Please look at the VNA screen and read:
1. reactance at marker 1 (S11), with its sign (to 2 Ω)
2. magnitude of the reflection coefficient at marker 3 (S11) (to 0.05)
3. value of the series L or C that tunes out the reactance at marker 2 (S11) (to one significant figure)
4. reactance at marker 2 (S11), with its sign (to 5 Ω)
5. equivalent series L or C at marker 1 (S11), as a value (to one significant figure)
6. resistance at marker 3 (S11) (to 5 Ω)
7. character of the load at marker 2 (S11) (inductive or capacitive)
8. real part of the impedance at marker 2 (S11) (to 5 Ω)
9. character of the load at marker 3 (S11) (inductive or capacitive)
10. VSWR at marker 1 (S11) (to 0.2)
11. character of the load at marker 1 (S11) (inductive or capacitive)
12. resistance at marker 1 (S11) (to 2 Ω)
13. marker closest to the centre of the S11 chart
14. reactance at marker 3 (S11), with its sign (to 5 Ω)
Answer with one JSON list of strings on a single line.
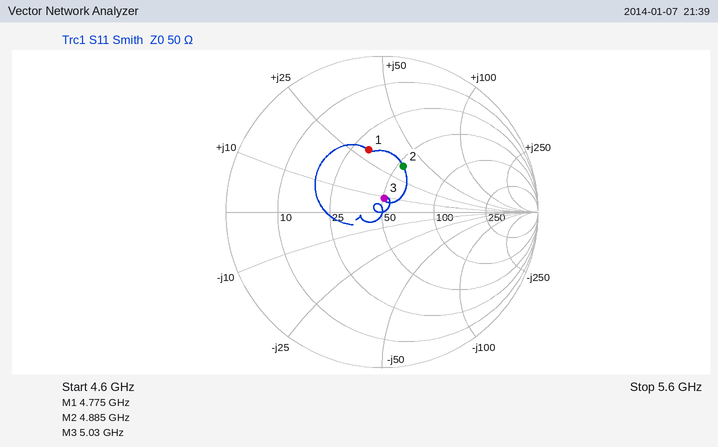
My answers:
["+30 Ω", "0.10", "900 fF", "+35 Ω", "1.0 nH", "50 Ω", "inductive", "55 Ω", "inductive", "2.4", "inductive", "32 Ω", "marker 3", "+10 Ω"]
